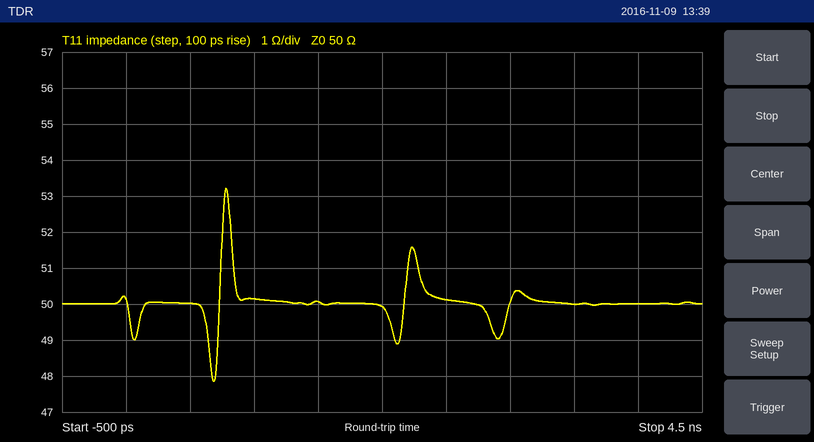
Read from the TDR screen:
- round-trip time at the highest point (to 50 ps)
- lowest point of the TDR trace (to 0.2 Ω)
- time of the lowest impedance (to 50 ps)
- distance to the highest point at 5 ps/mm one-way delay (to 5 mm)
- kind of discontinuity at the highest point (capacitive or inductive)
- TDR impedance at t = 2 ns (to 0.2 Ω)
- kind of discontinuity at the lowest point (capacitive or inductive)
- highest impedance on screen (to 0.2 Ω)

800 ps
47.8 Ω
700 ps
80 mm
inductive
50.0 Ω
capacitive
53.2 Ω
